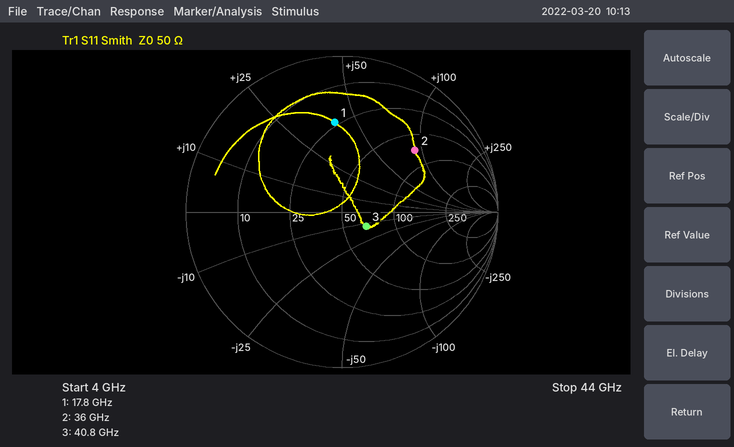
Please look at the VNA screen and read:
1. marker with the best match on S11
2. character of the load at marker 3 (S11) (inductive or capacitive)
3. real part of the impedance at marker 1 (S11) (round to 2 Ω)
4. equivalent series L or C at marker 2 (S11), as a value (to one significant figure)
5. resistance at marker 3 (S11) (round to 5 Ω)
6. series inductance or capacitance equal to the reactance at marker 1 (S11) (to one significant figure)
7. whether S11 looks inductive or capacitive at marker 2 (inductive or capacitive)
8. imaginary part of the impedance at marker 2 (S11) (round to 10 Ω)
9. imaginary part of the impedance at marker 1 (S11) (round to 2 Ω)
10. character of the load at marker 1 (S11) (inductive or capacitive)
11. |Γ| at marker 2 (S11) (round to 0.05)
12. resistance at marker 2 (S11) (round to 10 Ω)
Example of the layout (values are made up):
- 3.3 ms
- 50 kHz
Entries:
- marker 3
- capacitive
- 24 Ω
- 400 pH
- 65 Ω
- 400 pH
- inductive
- +90 Ω
- +40 Ω
- inductive
- 0.60
- 70 Ω
